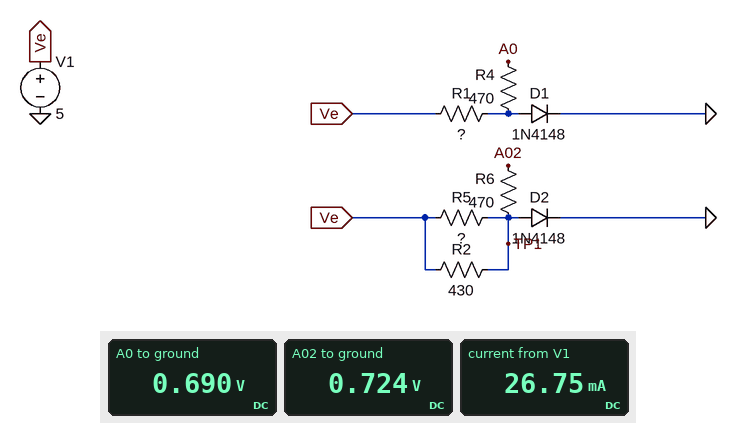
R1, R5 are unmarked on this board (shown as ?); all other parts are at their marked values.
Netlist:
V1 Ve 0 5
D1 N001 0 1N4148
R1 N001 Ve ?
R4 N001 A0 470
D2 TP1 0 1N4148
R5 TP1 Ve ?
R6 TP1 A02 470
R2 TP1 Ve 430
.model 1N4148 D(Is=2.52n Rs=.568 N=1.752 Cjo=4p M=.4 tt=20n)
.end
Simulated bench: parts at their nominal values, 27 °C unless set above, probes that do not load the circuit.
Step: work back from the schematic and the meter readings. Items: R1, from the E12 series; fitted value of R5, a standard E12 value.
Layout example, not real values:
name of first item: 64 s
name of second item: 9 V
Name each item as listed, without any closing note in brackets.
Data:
R1, from the E12 series: 470 Ω
fitted value of R5, a standard E12 value: 560 Ω
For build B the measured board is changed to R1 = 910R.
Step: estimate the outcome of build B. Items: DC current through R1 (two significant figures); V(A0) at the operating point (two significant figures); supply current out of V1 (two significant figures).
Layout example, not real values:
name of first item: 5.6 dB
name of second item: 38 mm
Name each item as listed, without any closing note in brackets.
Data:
DC current through R1: 4.8 mA
V(A0) at the operating point: 660 mV
supply current out of V1: 22 mA
